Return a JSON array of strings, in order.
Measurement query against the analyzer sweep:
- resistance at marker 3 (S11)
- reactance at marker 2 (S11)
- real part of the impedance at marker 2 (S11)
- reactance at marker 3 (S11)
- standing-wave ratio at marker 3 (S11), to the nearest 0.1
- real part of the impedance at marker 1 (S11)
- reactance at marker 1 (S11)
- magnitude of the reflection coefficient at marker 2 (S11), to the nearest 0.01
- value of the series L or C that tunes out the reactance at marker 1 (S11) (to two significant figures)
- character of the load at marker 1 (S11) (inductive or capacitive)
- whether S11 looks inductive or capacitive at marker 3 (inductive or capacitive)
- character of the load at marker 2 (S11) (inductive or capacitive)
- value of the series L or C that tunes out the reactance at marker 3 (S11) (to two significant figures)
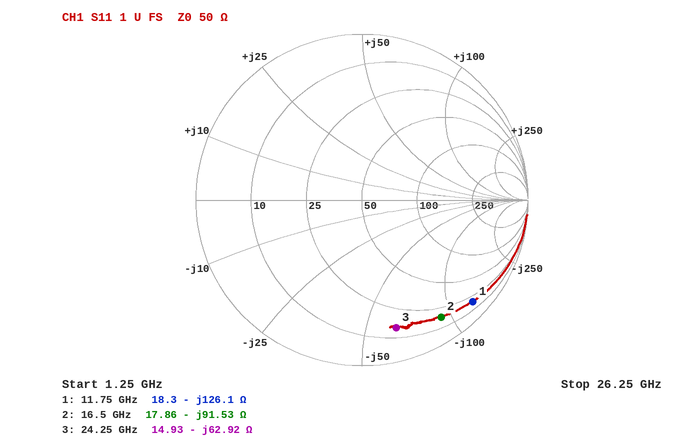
["14.93 Ω", "-91.53 Ω", "17.86 Ω", "-62.92 Ω", "8.8", "18.3 Ω", "-126.1 Ω", "0.85", "1.7 nH", "capacitive", "capacitive", "capacitive", "410 pH"]
